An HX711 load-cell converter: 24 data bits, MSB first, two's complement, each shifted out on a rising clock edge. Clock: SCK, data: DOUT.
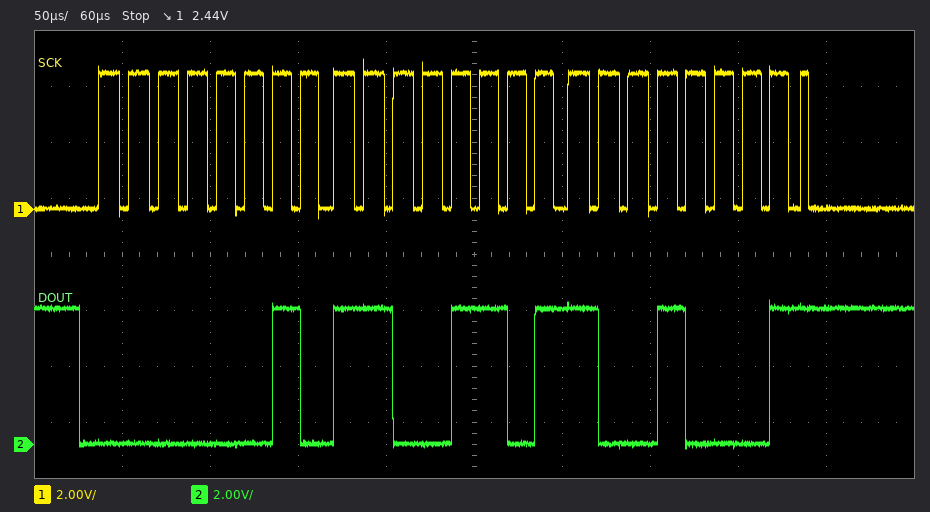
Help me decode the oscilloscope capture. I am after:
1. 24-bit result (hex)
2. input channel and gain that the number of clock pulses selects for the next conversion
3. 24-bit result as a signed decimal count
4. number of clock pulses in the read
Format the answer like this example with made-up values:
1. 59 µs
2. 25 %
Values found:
1. 0x02CD91
2. channel A, gain 128
3. 183697
4. 25
